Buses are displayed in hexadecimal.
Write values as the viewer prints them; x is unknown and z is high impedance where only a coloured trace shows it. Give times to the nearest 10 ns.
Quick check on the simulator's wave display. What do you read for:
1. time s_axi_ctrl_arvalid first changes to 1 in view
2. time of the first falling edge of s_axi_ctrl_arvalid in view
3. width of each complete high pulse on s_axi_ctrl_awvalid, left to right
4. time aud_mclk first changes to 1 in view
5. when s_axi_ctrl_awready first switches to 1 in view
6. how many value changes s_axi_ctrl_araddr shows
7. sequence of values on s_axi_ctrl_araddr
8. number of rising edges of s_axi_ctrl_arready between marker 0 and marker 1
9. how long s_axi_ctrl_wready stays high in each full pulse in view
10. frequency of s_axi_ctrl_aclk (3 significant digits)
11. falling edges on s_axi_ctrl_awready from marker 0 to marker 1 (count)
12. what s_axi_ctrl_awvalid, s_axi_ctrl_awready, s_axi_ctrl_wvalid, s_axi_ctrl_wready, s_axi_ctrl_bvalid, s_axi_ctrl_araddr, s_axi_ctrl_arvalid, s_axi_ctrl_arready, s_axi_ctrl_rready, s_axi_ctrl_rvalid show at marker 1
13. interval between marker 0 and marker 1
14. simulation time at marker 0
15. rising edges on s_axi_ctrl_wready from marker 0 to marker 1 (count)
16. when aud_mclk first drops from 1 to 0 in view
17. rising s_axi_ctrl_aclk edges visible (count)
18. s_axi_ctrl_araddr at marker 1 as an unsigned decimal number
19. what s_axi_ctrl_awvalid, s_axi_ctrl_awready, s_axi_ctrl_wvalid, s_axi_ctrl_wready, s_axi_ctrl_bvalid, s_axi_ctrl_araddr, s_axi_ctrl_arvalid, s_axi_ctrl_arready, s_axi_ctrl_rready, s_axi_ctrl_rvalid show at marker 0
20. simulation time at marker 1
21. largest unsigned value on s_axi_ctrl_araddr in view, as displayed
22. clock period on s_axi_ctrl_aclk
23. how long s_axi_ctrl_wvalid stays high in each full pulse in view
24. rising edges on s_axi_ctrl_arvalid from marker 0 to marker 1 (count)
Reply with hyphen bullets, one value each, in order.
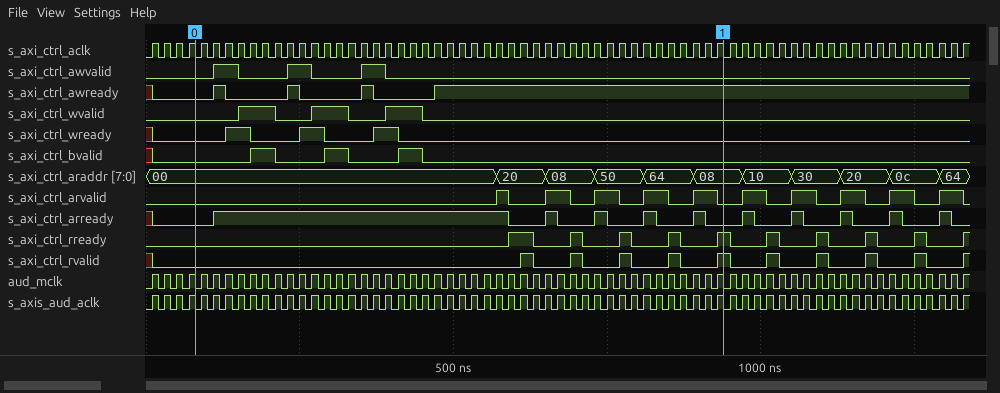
- 570 ns
- 590 ns
- 40 ns, 40 ns, 40 ns
- 10 ns
- 110 ns
- 10
- 00, 20, 08, 50, 64, 08, 10, 30, 20, 0c, 64
- 5
- 40 ns, 40 ns, 40 ns
- 50.0 MHz
- 3
- s_axi_ctrl_awvalid=0, s_axi_ctrl_awready=1, s_axi_ctrl_wvalid=0, s_axi_ctrl_wready=0, s_axi_ctrl_bvalid=0, s_axi_ctrl_araddr=08, s_axi_ctrl_arvalid=0, s_axi_ctrl_arready=0, s_axi_ctrl_rready=1, s_axi_ctrl_rvalid=1
- 860 ns
- 80 ns
- 3
- 20 ns
- 67
- 8
- s_axi_ctrl_awvalid=0, s_axi_ctrl_awready=0, s_axi_ctrl_wvalid=0, s_axi_ctrl_wready=0, s_axi_ctrl_bvalid=0, s_axi_ctrl_araddr=00, s_axi_ctrl_arvalid=0, s_axi_ctrl_arready=0, s_axi_ctrl_rready=0, s_axi_ctrl_rvalid=0
- 940 ns
- 64
- 20 ns
- 60 ns, 60 ns, 60 ns
- 5
